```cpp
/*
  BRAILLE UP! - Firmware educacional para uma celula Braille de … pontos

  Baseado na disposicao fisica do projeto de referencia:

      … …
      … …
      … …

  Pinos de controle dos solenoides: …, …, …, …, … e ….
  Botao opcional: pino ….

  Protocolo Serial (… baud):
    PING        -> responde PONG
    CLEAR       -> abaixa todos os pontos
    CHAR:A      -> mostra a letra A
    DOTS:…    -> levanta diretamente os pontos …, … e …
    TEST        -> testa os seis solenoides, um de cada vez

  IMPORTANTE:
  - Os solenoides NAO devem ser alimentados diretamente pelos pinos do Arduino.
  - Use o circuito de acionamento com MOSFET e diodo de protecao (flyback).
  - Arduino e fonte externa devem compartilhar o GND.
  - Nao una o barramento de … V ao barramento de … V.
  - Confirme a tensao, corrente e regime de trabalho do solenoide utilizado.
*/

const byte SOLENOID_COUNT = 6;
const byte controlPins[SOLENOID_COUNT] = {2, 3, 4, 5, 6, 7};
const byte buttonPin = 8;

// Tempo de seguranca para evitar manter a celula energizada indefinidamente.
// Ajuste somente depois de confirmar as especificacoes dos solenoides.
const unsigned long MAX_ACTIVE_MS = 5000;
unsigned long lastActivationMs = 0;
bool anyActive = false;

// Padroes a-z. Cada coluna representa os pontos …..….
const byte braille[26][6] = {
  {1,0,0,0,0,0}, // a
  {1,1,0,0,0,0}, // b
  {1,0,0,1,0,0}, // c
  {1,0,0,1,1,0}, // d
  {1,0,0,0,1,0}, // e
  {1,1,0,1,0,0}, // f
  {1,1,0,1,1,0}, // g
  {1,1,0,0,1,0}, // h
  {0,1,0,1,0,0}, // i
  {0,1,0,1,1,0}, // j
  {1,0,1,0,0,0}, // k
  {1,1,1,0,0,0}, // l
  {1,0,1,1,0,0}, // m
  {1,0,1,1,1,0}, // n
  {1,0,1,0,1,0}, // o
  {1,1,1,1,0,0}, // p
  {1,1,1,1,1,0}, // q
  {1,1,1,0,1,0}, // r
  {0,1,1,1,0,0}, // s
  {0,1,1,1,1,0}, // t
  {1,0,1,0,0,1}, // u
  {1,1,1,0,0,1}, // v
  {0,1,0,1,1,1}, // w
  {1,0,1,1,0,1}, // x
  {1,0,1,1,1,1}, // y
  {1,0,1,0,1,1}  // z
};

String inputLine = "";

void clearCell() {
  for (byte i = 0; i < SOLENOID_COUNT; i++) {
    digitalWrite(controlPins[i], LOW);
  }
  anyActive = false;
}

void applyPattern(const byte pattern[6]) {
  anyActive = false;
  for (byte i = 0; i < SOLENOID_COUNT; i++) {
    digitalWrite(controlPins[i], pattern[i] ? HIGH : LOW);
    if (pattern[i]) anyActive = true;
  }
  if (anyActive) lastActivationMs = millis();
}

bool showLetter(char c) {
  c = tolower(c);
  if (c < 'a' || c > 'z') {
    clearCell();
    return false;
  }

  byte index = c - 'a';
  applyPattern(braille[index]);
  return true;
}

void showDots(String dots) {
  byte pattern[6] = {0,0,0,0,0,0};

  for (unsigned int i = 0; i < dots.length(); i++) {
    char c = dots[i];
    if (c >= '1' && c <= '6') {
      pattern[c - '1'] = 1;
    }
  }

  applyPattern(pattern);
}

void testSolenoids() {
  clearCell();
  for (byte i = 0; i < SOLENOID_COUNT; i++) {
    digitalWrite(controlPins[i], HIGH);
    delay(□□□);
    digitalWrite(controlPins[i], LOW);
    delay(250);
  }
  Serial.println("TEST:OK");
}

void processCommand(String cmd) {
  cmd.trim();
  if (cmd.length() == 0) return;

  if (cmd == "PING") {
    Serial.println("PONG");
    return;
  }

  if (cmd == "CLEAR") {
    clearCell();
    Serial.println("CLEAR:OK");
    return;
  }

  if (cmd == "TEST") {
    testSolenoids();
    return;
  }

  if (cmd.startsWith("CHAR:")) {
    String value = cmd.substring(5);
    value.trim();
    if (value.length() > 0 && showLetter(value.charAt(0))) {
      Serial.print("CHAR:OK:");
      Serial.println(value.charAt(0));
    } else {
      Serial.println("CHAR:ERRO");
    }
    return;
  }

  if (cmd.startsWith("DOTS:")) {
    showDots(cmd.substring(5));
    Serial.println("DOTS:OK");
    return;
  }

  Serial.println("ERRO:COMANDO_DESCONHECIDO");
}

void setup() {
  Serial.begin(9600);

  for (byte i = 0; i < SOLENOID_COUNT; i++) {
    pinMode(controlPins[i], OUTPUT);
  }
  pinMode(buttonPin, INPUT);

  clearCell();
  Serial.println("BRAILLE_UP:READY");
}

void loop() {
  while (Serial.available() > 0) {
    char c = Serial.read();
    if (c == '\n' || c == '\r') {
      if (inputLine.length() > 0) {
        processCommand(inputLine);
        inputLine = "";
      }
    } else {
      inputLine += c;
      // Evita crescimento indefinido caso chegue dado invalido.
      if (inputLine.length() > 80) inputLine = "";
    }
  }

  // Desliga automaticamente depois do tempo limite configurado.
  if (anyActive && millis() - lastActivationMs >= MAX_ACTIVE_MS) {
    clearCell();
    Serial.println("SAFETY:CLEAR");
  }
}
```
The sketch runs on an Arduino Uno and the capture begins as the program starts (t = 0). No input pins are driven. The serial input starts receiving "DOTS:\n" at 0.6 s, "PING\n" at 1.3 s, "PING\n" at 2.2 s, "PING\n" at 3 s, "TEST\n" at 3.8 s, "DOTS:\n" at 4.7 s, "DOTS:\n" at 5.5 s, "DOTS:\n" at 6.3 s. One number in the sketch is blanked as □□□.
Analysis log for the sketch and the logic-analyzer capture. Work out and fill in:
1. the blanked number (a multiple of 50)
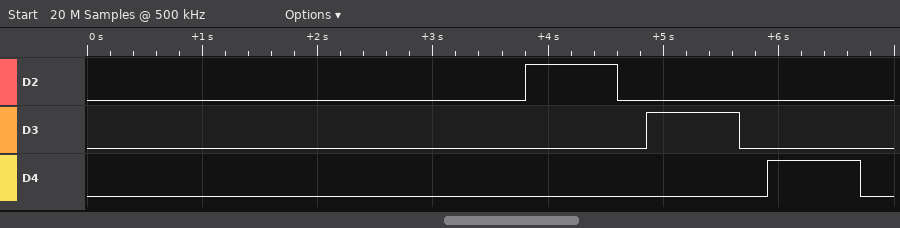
800
